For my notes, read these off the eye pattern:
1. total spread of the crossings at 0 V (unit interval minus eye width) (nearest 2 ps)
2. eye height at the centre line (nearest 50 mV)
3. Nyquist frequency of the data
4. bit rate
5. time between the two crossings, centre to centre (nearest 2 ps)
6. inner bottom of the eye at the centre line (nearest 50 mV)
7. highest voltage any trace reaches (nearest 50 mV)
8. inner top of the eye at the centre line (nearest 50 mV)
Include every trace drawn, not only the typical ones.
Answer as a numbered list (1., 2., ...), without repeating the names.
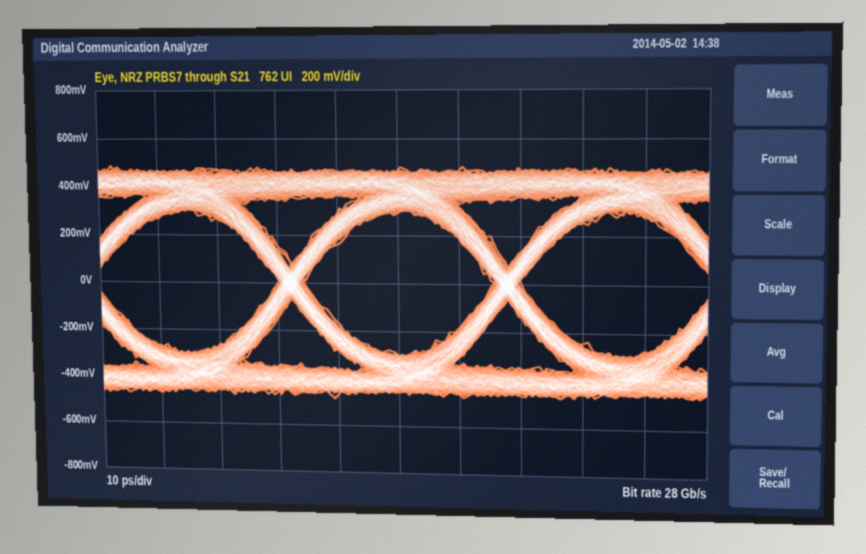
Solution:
1. 4 ps
2. 600 mV
3. 14 GHz
4. 28 Gb/s
5. 36 ps
6. -300 mV
7. 500 mV
8. 300 mV
